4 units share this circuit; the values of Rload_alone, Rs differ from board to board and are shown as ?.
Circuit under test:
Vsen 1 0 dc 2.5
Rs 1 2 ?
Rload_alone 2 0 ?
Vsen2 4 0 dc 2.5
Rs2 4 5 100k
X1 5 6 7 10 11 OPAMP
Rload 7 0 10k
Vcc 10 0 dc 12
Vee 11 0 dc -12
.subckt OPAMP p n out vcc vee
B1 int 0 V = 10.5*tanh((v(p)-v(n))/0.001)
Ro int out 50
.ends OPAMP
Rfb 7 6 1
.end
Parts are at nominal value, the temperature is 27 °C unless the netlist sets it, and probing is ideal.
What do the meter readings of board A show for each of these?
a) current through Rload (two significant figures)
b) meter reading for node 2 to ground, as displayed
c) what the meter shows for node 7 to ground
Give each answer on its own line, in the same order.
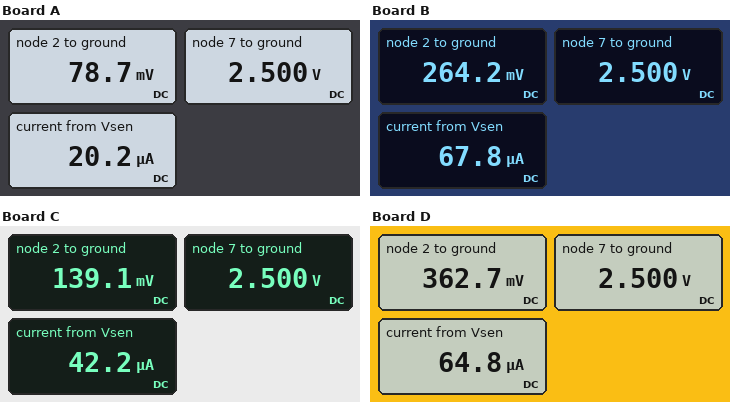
250 µA
78.7 mV
2.500 V
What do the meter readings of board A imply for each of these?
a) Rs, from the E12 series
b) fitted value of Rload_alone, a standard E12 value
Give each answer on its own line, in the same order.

120 kΩ
3.9 kΩ
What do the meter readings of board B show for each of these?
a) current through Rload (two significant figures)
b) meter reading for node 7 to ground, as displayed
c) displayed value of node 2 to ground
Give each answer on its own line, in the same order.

250 µA
2.500 V
264.2 mV
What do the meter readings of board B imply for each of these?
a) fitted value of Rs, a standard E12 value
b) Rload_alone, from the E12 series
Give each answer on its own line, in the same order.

33 kΩ
3.9 kΩ
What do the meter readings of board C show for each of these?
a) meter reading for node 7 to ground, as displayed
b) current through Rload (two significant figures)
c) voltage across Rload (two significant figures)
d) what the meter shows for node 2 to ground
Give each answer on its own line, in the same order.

2.500 V
250 µA
2.5 V
139.1 mV
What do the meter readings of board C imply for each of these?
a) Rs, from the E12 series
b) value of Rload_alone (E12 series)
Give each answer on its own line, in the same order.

56 kΩ
3.3 kΩ
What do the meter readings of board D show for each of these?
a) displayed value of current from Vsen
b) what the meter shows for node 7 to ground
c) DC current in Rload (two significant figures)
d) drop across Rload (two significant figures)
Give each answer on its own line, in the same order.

64.8 µA
2.500 V
250 µA
2.5 V
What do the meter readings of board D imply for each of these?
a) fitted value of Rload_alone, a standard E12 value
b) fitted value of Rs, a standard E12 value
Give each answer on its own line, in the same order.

5.6 kΩ
33 kΩ
